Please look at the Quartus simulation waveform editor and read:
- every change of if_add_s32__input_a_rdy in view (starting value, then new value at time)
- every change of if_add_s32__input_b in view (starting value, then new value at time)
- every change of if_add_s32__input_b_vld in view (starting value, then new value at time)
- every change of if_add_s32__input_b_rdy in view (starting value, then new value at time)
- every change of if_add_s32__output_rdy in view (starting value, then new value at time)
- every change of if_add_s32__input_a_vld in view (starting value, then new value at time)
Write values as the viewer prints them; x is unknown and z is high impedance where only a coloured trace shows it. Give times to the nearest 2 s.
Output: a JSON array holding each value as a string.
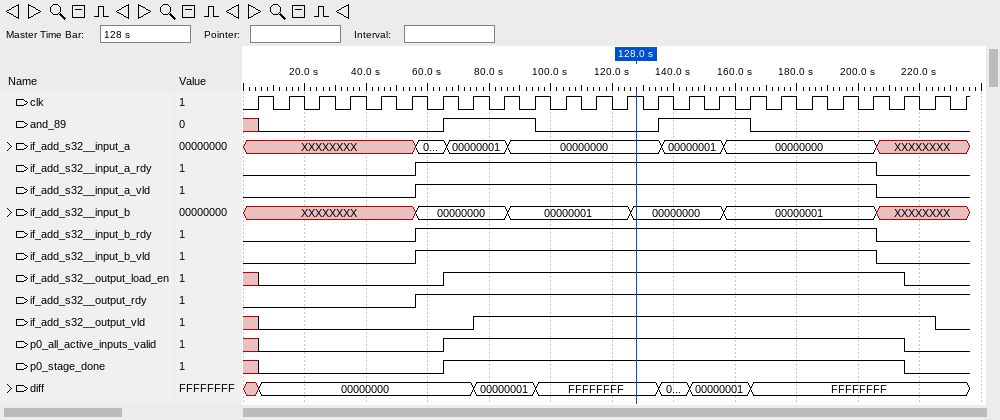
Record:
["0, 1 at 56 s, 0 at 206 s", "XXXXXXXX, 00000000 at 56 s, 00000001 at 86 s, 00000000 at 126 s, 00000001 at 156 s, XXXXXXXX at 206 s", "0, 1 at 56 s, 0 at 206 s", "0, 1 at 56 s, 0 at 206 s", "0, 1 at 56 s", "0, 1 at 56 s, 0 at 206 s"]
